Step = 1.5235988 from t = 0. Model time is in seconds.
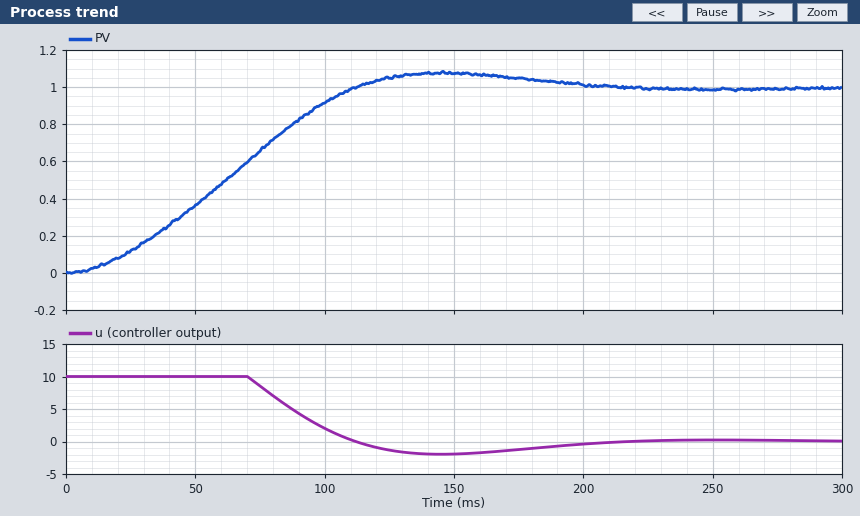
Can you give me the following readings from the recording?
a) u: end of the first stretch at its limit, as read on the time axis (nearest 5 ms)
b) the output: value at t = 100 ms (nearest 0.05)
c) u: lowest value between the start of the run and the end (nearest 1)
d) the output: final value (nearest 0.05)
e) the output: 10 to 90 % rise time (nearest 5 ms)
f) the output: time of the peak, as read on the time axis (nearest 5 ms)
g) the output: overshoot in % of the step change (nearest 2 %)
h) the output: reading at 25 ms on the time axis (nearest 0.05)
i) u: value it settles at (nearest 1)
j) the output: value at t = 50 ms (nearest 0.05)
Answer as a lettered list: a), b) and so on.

a) 70 ms
b) 0.90
c) -2
d) 1.00
e) 75 ms
f) 145 ms
g) 8 %
h) 0.10
i) 0
j) 0.35
